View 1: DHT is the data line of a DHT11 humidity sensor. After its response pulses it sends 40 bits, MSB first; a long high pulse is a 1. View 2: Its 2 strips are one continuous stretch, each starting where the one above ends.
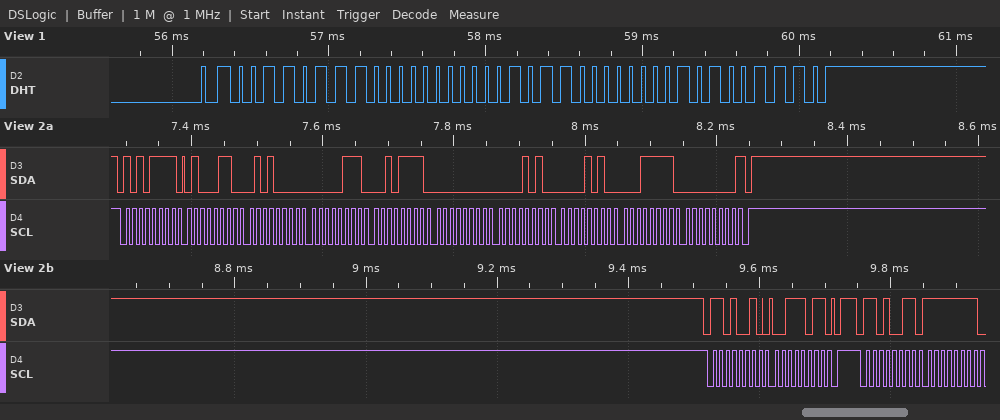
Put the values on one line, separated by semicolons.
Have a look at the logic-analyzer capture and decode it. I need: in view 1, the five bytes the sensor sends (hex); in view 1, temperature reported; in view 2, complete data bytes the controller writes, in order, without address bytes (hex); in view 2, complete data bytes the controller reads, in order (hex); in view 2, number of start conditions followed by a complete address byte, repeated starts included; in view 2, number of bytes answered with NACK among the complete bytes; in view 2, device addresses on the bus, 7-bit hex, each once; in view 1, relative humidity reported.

37 00 16 01 4E; 22.1 °C; 3B; 46 50 07 2F 00 0A 0A 1F 00 FF; 3; 1; 0x57 0x69; 55 %
